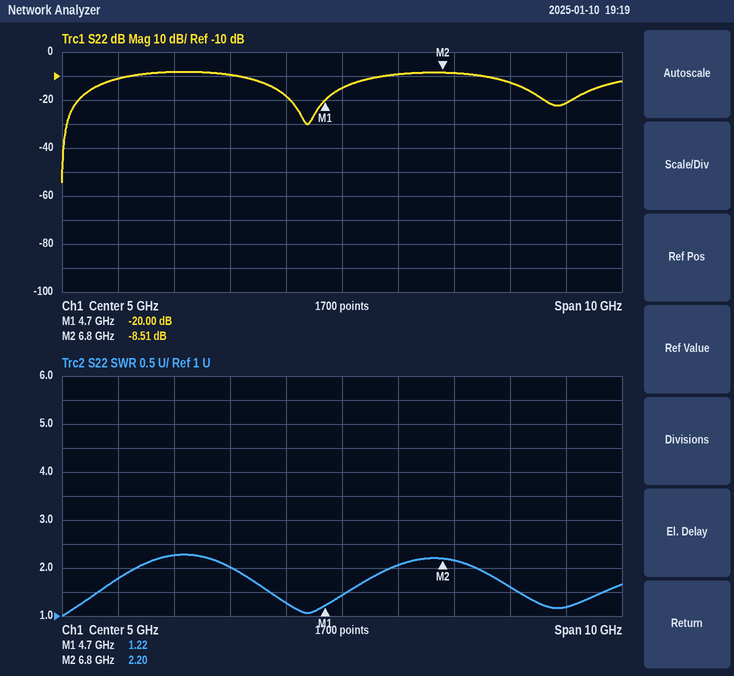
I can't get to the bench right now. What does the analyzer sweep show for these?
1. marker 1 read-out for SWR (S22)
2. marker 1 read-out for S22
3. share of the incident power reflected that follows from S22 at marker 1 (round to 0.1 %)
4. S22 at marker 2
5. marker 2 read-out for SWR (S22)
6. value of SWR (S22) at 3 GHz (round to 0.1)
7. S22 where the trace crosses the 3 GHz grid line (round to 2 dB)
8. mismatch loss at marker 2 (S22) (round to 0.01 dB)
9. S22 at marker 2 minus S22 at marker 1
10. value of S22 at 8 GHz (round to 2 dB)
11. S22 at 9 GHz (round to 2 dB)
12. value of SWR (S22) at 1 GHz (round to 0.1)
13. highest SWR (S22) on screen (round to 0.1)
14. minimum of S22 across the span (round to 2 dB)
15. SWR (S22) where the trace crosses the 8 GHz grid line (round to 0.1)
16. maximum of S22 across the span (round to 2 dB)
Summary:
1.22
-20.00 dB
1.0 %
-8.51 dB
2.20
2.0
-10 dB
0.66 dB
11.49 dB
-12 dB
-22 dB
1.8
2.3
-54 dB
1.6
-8 dB
